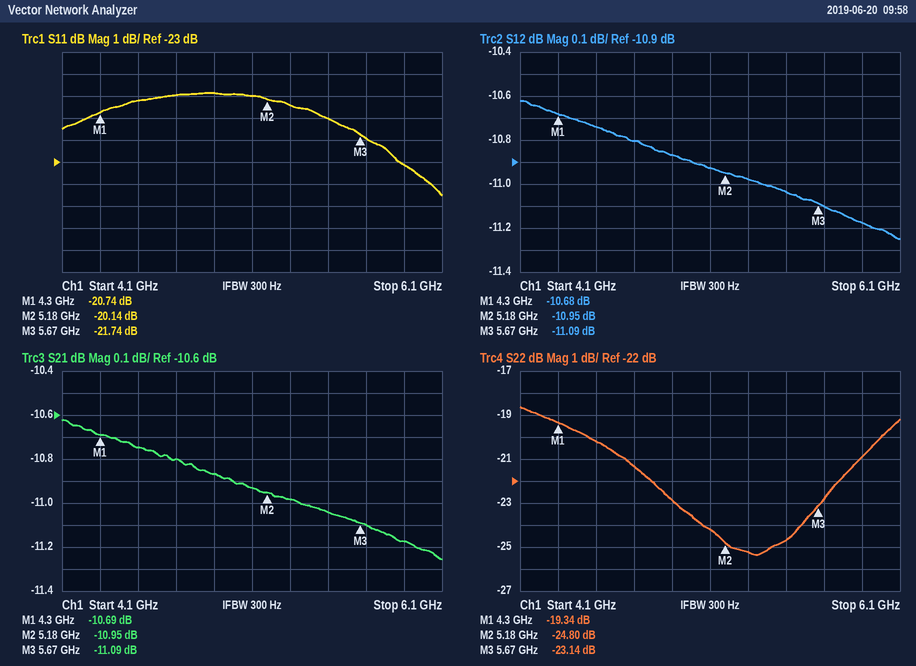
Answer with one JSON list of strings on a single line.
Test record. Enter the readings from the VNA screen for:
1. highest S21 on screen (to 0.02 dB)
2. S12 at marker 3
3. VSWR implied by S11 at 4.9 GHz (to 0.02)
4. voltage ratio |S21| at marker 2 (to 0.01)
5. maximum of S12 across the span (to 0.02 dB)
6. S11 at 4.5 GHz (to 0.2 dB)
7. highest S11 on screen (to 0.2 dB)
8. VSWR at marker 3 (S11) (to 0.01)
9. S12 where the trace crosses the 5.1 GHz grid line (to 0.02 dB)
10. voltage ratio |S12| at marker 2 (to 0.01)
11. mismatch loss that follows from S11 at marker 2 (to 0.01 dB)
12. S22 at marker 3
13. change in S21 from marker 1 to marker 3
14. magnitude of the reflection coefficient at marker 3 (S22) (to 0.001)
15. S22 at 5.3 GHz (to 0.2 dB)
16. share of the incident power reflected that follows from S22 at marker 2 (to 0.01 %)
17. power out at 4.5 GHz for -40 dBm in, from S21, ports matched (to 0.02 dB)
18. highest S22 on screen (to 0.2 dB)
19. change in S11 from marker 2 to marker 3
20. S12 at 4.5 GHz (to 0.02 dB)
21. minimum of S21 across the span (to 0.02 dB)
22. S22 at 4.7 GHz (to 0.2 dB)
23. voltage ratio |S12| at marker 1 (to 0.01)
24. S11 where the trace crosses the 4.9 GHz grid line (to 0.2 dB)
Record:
["-10.62 dB", "-11.09 dB", "1.22", "0.28", "-10.62 dB", "-20.2 dB", "-19.8 dB", "1.18", "-10.92 dB", "0.28", "0.04 dB", "-23.14 dB", "-0.40 dB", "0.070", "-25.2 dB", "0.33 %", "-50.74 dBm", "-18.6 dB", "-1.60 dB", "-10.74 dB", "-11.26 dB", "-21.4 dB", "0.29", "-19.8 dB"]
